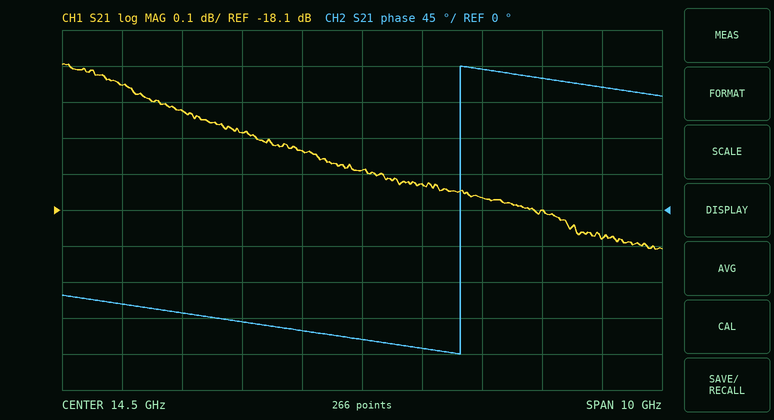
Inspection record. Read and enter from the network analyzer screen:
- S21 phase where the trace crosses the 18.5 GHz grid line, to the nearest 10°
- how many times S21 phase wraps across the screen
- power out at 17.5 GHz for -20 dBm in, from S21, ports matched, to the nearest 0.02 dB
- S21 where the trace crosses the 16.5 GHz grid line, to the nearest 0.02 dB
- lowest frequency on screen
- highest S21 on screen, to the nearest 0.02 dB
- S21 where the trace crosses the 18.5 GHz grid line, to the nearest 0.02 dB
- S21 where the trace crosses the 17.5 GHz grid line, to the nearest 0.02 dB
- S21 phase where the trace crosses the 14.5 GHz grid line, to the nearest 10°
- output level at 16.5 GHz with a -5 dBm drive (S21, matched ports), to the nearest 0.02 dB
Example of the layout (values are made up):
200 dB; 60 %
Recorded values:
150°; 1; -38.10 dBm; -18.06 dB; 9.5 GHz; -17.70 dB; -18.18 dB; -18.10 dB; -160°; -23.06 dBm
